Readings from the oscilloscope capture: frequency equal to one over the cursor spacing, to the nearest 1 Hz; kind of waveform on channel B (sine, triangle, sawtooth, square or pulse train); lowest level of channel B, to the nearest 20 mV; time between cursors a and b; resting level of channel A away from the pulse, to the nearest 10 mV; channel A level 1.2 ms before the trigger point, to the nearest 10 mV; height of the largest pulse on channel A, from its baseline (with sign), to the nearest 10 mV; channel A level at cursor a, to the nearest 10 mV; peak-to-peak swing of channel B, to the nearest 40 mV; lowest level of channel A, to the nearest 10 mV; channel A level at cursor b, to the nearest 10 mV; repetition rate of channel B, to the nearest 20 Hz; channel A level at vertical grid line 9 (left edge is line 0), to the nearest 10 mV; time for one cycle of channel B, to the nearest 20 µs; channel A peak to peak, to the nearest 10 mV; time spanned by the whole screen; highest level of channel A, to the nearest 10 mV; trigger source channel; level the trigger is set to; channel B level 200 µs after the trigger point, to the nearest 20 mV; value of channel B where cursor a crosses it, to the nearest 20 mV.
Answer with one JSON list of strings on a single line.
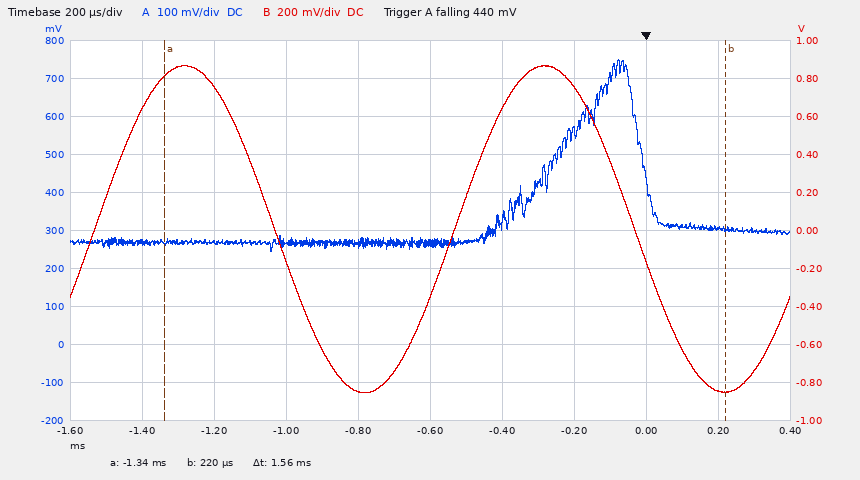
["641 Hz", "sine", "-860 mV", "1.56 ms", "270 mV", "270 mV", "+480 mV", "270 mV", "1.72 V", "240 mV", "300 mV", "1.00 kHz", "310 mV", "1.00 ms", "510 mV", "2 ms", "750 mV", "channel A", "440 mV", "-840 mV", "820 mV"]
